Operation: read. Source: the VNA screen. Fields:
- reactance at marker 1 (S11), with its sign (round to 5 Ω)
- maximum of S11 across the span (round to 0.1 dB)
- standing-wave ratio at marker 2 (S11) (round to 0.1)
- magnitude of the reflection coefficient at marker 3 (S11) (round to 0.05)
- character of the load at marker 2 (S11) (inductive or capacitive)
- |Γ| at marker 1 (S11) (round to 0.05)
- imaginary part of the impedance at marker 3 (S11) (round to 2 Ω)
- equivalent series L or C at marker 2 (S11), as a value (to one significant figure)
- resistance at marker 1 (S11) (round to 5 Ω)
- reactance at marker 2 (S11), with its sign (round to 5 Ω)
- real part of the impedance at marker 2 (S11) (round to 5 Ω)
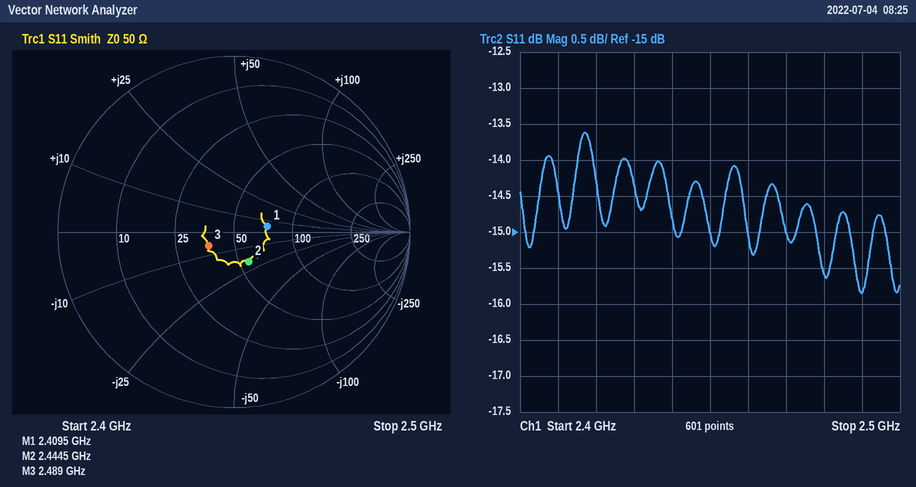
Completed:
+5 Ω
-13.6 dB
1.5
0.15
capacitive
0.20
-6 Ω
3 pF
75 Ω
-20 Ω
55 Ω
